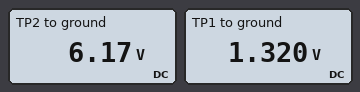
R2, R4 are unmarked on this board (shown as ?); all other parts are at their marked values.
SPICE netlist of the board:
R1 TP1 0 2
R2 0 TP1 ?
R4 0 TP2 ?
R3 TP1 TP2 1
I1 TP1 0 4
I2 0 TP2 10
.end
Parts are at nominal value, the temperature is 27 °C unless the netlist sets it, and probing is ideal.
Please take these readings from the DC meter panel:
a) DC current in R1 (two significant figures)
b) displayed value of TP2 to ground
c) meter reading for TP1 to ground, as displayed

660 mA
6.17 V
1.320 V
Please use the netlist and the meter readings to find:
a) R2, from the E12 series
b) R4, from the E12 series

6.8 Ω
1.2 Ω
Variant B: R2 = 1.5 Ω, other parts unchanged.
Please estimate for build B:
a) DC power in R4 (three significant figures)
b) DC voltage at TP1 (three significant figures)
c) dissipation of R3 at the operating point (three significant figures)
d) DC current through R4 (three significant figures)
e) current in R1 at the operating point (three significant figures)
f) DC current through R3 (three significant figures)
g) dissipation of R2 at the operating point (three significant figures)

29.4 W
897 mV
25.5 W
4.95 A
449 mA
5.05 A
537 mW
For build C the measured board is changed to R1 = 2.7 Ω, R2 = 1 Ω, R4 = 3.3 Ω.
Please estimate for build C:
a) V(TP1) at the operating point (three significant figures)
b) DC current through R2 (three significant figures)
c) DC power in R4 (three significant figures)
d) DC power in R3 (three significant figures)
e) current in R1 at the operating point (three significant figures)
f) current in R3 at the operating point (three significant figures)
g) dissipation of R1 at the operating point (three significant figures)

2.29 V
2.29 A
27.0 W
51.0 W
849 mA
7.14 A
1.95 W
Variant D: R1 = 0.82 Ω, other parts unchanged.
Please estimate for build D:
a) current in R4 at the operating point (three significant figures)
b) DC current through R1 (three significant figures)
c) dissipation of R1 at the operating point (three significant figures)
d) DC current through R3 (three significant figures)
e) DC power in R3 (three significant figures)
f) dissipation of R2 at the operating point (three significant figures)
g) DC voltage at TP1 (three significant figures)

4.91 A
974 mA
778 mW
5.09 A
25.9 W
93.8 mW
799 mV
